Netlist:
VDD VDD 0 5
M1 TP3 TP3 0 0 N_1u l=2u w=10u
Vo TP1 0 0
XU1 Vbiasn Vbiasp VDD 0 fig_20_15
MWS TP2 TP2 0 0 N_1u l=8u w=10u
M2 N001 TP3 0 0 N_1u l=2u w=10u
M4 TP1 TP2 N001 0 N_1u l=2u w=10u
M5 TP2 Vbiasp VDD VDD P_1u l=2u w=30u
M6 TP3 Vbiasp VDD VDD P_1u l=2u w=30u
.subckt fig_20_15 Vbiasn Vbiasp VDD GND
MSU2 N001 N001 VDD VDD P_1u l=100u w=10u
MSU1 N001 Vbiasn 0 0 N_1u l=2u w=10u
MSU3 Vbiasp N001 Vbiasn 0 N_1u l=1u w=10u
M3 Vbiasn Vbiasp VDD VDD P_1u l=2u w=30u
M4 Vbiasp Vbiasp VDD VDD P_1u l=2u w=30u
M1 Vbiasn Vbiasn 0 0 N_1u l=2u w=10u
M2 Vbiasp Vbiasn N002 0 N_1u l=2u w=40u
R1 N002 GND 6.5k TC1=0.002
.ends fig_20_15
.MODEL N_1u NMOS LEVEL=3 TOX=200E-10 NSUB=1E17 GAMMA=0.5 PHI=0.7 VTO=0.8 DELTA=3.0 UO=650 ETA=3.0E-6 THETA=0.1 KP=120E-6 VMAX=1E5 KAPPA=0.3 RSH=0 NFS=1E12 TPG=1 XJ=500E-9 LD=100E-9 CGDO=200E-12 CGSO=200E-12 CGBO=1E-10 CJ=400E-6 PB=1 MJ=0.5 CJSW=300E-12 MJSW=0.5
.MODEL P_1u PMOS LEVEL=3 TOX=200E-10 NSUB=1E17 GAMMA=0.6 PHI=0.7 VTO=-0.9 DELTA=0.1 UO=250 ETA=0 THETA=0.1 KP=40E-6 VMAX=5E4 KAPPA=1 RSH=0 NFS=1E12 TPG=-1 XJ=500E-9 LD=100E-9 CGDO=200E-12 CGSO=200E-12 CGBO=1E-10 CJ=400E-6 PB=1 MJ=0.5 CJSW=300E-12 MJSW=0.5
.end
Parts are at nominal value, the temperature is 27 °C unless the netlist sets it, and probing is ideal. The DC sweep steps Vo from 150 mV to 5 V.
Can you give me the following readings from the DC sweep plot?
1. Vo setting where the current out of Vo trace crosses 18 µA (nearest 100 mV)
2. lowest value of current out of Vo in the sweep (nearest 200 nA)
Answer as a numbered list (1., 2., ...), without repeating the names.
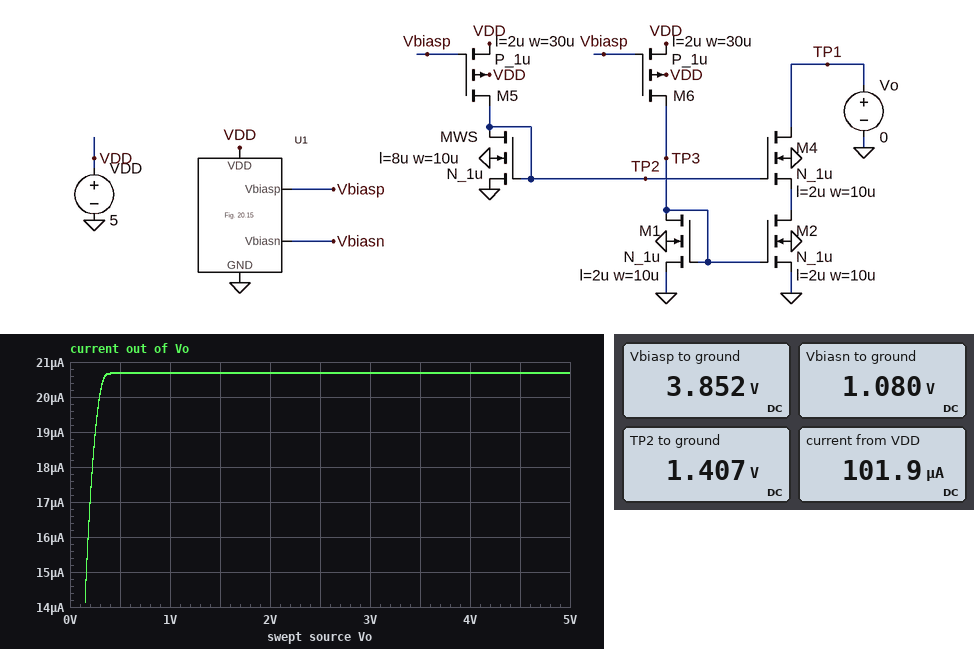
1. 200 mV
2. 14.2 µA
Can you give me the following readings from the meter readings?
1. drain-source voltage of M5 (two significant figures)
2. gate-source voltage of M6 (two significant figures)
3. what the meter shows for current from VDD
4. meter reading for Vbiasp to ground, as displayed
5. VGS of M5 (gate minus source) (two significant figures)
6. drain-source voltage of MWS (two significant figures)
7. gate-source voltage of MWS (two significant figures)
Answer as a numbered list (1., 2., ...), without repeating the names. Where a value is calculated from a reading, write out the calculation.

1. 1.407 V - 5 V = -3.6 V
2. 3.852 V - 5 V = -1.1 V
3. 101.9 µA
4. 3.852 V
5. 3.852 V - 5 V = -1.1 V
6. 1.407 V = 1.4 V
7. 1.407 V = 1.4 V
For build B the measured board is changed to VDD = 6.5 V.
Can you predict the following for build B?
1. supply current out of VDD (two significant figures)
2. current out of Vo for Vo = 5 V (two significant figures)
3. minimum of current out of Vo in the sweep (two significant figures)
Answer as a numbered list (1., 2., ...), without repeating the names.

1. 110 µA
2. 22 µA
3. 15 µA
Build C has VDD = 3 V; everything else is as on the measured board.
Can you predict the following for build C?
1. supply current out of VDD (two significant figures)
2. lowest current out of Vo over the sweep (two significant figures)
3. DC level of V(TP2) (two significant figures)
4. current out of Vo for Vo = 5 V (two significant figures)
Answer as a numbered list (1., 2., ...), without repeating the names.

1. 83 µA
2. 13 µA
3. 1.4 V
4. 19 µA
